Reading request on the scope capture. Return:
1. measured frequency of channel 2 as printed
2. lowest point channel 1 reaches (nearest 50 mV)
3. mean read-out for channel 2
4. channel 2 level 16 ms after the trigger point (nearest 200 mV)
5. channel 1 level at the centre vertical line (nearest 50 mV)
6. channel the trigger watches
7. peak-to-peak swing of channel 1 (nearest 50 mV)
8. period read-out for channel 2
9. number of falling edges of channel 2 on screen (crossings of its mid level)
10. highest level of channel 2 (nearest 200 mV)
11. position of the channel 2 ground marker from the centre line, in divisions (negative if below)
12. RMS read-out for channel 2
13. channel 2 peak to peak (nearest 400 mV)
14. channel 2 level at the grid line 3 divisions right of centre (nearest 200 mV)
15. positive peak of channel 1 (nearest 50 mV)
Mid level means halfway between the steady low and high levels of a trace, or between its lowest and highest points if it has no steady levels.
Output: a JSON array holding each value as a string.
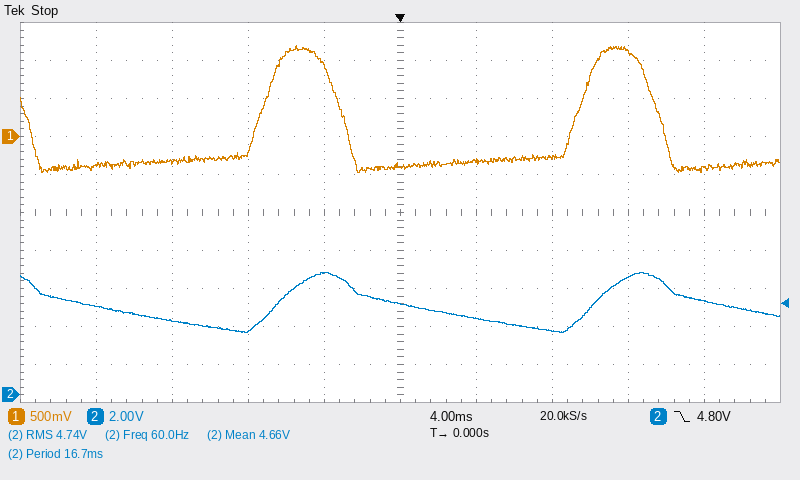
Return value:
["60.0 Hz", "-450 mV", "4.66 V", "5.0 V", "-400 mV", "channel 2", "1.65 V", "16.7 ms", "3", "6.4 V", "-4.8 div", "4.74 V", "3.2 V", "6.2 V", "1.20 V"]
